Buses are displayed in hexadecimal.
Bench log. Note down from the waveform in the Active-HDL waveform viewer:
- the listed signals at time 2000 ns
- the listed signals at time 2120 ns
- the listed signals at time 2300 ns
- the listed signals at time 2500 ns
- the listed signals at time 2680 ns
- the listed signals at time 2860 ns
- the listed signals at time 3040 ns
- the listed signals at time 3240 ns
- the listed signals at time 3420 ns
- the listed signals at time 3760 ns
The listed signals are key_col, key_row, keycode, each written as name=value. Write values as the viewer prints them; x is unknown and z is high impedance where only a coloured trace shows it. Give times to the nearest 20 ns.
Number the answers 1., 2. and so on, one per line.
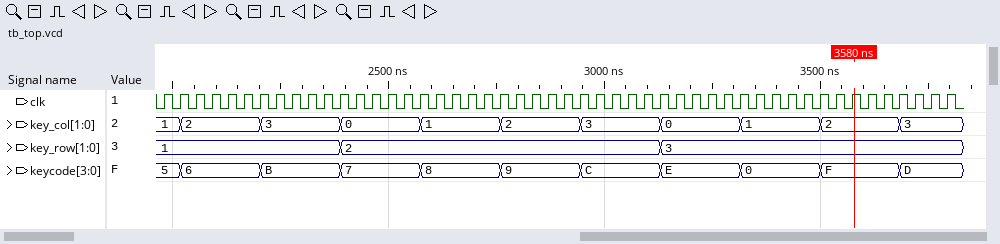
1. key_col=1, key_row=1, keycode=5
2. key_col=2, key_row=1, keycode=6
3. key_col=3, key_row=1, keycode=B
4. key_col=0, key_row=2, keycode=7
5. key_col=1, key_row=2, keycode=8
6. key_col=2, key_row=2, keycode=9
7. key_col=3, key_row=2, keycode=C
8. key_col=0, key_row=3, keycode=E
9. key_col=1, key_row=3, keycode=0
10. key_col=3, key_row=3, keycode=D
